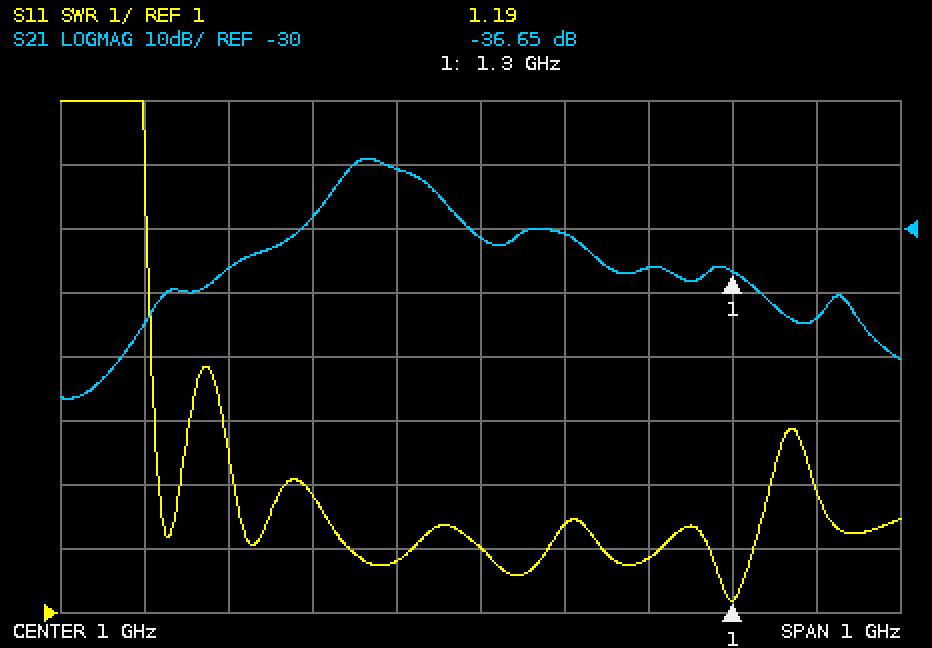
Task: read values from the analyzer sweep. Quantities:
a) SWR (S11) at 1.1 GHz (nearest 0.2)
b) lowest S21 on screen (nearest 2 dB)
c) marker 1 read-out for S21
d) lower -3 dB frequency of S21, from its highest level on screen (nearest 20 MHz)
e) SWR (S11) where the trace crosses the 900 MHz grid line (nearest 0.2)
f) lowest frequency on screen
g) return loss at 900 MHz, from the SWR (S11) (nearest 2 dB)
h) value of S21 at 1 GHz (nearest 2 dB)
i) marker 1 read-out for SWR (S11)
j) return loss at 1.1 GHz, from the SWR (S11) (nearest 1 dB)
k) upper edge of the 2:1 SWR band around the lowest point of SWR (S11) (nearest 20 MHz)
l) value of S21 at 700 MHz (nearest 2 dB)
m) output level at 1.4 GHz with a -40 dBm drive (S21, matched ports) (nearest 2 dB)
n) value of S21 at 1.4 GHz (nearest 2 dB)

2.4
-56 dB
-36.65 dB
840 MHz
1.8
500 MHz
10 dB
-32 dB
1.19
8 dB
1.32 GHz
-36 dB
-84 dBm
-44 dB
